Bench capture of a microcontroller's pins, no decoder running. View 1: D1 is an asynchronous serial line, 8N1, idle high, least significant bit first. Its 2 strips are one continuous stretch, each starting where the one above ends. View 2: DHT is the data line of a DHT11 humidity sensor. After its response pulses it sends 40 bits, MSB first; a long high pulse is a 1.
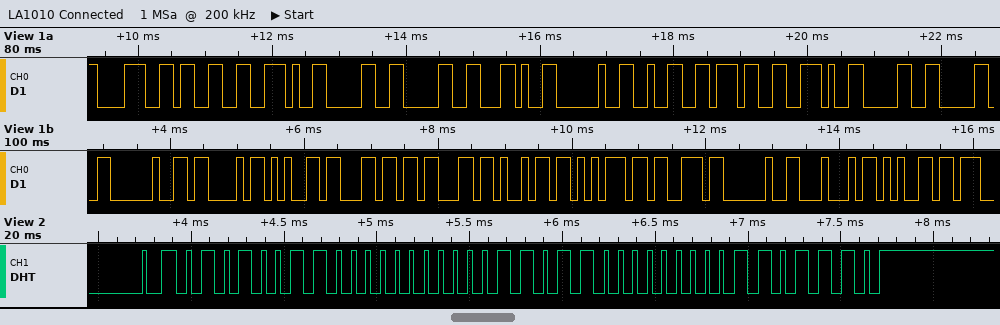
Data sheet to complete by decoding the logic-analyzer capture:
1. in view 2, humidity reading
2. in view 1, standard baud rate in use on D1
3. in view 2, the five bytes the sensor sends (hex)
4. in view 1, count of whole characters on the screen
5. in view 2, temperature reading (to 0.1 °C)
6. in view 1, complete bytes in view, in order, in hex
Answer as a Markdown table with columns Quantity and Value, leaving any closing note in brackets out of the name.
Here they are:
| Quantity | Value |
|---|---|
| in view 2, humidity reading | 83 % |
| in view 1, standard baud rate in use on D1 | 9600 baud |
| in view 2, the five bytes the sensor sends | 53 00 1B 00 6E |
| in view 1, count of whole characters on the screen | 23 |
| in view 2, temperature reading | 27.0 °C |
| in view 1, complete bytes in view, in order, in hex | 0x38 0x33 0x2E 0x30 0x30 0x2C 0x20 0x32 0x37 0x2E 0x30 0x30 0x20 0x43 0x65 0x6C 0x63 0x69 0x75 0x73 0x20 0x44 0x65 |
